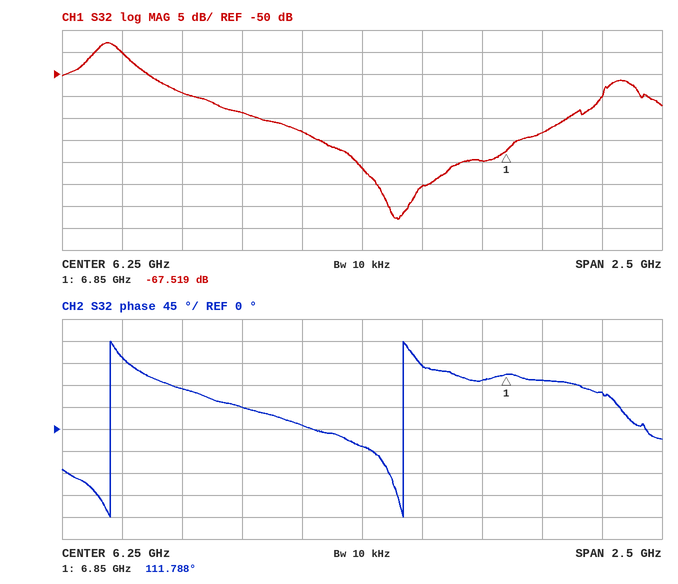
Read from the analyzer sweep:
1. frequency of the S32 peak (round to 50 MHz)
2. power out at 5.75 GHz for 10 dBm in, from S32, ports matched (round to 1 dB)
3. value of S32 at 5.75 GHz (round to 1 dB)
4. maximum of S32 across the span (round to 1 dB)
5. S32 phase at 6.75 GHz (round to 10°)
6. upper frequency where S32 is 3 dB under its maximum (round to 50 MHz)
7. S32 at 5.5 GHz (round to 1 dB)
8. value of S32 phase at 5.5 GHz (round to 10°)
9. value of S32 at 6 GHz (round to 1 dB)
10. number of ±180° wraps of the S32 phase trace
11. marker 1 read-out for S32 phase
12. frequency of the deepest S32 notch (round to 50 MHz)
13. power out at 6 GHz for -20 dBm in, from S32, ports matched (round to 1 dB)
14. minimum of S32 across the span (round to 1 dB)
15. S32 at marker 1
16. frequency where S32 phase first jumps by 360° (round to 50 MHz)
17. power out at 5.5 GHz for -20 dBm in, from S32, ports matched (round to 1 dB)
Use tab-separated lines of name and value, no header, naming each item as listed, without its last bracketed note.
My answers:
frequency of the S32 peak	5.20 GHz
power out at 5.75 GHz for 10 dBm in, from S32, ports matched	-49 dBm
value of S32 at 5.75 GHz	-59 dB
maximum of S32 across the span	-43 dB
S32 phase at 6.75 GHz	100°
upper frequency where S32 is 3 dB under its maximum	5.25 GHz
S32 at 5.5 GHz	-54 dB
value of S32 phase at 5.5 GHz	80°
value of S32 at 6 GHz	-63 dB
number of ±180° wraps of the S32 phase trace	2
marker 1 read-out for S32 phase	111.788°
frequency of the deepest S32 notch	6.40 GHz
power out at 6 GHz for -20 dBm in, from S32, ports matched	-83 dBm
minimum of S32 across the span	-83 dB
S32 at marker 1	-67.519 dB
frequency where S32 phase first jumps by 360°	5.20 GHz
power out at 5.5 GHz for -20 dBm in, from S32, ports matched	-74 dBm
